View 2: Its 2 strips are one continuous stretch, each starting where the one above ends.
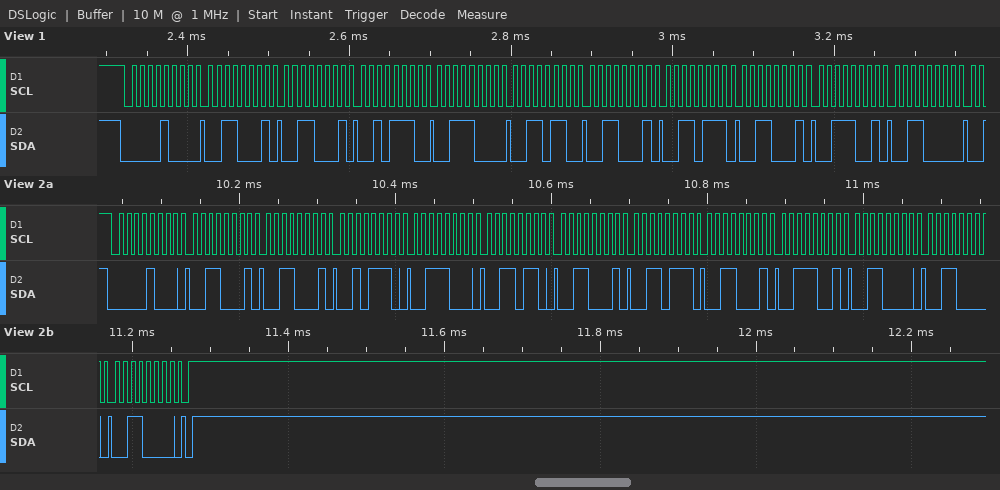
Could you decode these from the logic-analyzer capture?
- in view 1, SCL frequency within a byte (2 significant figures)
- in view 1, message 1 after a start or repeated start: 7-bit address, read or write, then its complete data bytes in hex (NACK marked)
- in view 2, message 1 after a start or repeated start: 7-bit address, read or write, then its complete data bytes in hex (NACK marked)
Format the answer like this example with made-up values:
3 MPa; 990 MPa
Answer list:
100 kHz; 0x04 write: 31 31 2E 38 36 31 37 31 39 30; 0x04 write: 31 31 2E 38 36 31 37 31 39 30 30 30
